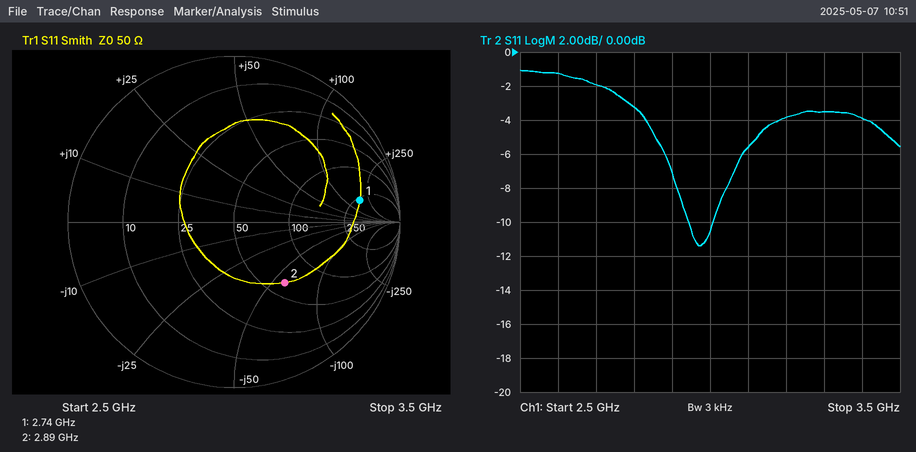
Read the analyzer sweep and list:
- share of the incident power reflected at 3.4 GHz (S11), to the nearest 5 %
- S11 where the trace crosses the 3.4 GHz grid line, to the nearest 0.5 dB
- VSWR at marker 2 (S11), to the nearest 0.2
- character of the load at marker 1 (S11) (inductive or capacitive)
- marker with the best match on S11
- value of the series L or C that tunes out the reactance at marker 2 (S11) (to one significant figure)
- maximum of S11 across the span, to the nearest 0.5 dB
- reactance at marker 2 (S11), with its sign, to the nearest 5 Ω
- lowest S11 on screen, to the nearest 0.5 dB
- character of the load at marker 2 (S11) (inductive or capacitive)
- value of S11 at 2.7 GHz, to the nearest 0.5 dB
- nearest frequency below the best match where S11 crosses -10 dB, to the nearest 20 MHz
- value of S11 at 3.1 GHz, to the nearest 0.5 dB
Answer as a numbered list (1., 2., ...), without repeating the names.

1. 40 %
2. -4.0 dB
3. 2.8
4. inductive
5. marker 2
6. 3 nH
7. -1.0 dB
8. -60 Ω
9. -11.5 dB
10. capacitive
11. -2.0 dB
12. 2.94 GHz
13. -5.5 dB
